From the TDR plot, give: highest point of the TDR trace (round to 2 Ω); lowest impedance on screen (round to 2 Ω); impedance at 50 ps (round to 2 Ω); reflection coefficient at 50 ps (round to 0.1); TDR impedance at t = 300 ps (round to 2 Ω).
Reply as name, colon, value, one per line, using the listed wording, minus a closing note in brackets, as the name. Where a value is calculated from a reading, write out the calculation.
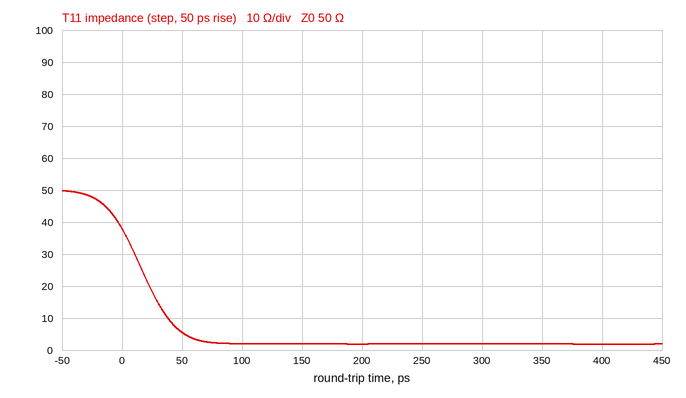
highest point of the TDR trace: 50 Ω
lowest impedance on screen: 2 Ω
impedance at 50 ps: 6 Ω
reflection coefficient at 50 ps: (6 − 50)/(6 + 50) ≈ -0.8
TDR impedance at t = 300 ps: 2 Ω
